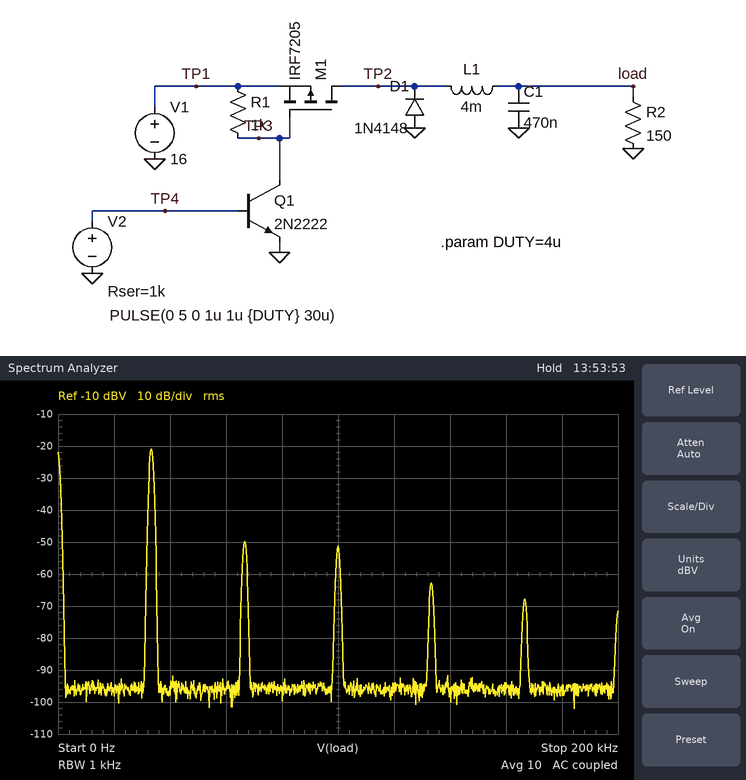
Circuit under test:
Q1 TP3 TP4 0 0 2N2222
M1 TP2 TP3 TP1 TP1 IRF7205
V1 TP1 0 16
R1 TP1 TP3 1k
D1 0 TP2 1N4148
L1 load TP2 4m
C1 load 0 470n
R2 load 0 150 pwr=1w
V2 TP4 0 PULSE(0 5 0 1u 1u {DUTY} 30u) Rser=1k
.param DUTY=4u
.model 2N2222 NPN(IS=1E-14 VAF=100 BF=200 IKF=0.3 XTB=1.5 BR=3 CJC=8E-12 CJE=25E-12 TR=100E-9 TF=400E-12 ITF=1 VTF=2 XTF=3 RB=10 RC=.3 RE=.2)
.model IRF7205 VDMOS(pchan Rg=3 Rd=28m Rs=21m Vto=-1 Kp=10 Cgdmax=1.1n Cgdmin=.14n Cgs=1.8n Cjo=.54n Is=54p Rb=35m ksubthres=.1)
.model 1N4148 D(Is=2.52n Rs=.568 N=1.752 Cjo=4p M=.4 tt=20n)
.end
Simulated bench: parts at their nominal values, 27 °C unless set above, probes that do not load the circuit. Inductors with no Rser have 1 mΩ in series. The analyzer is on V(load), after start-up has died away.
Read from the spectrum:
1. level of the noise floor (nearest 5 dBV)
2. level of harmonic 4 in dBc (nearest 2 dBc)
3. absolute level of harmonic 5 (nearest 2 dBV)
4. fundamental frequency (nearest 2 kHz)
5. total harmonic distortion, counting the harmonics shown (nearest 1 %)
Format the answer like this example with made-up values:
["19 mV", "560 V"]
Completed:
["-95 dBV", "-42 dBc", "-68 dBV", "34 kHz", "5 %"]
